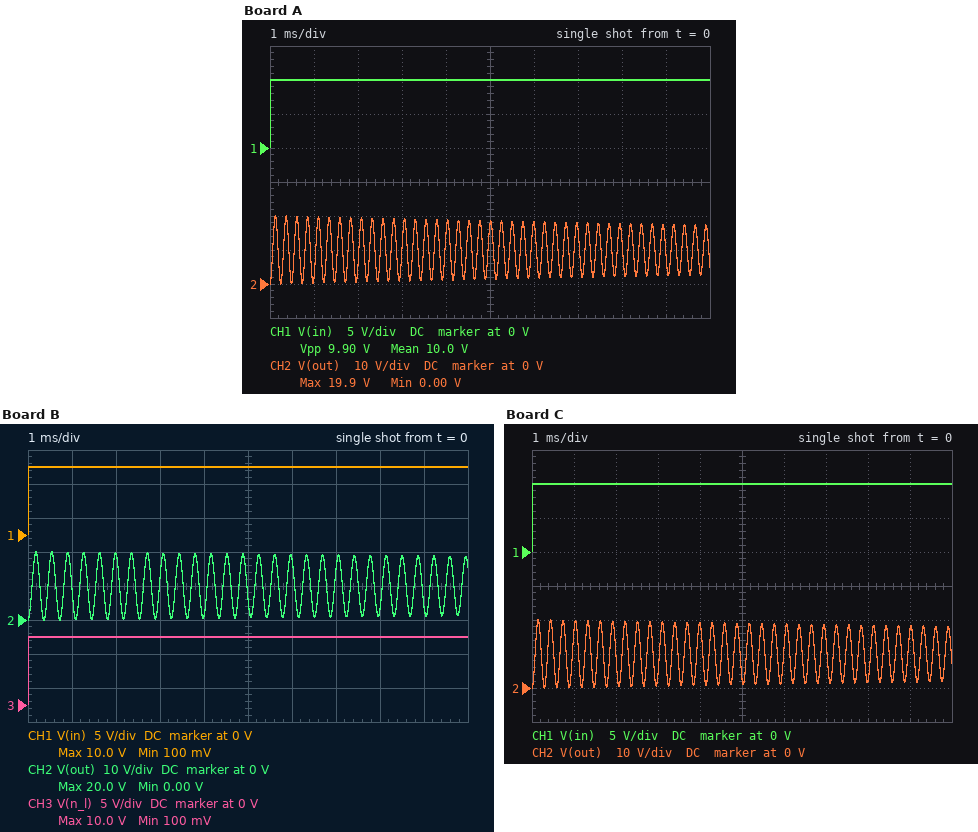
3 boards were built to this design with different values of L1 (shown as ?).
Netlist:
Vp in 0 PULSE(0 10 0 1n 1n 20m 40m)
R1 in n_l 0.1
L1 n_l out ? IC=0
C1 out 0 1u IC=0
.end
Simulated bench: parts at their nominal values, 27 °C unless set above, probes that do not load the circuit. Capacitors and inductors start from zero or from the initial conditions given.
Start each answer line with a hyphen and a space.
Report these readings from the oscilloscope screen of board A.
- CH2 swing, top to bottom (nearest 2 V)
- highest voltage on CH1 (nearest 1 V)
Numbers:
- 20 V
- 10 V
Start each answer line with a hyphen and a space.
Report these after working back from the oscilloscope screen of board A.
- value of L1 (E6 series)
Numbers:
- 1.5 mH
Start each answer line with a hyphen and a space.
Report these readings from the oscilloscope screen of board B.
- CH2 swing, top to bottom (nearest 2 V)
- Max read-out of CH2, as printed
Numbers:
- 20 V
- 20.0 V
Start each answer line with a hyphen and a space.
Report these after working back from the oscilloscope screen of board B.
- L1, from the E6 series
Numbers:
- 3.3 mH
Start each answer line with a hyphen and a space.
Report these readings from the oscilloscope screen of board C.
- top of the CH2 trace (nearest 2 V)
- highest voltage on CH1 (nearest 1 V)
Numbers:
- 20 V
- 10 V
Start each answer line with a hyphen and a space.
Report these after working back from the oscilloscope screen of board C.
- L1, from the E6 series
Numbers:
- 2.2 mH
